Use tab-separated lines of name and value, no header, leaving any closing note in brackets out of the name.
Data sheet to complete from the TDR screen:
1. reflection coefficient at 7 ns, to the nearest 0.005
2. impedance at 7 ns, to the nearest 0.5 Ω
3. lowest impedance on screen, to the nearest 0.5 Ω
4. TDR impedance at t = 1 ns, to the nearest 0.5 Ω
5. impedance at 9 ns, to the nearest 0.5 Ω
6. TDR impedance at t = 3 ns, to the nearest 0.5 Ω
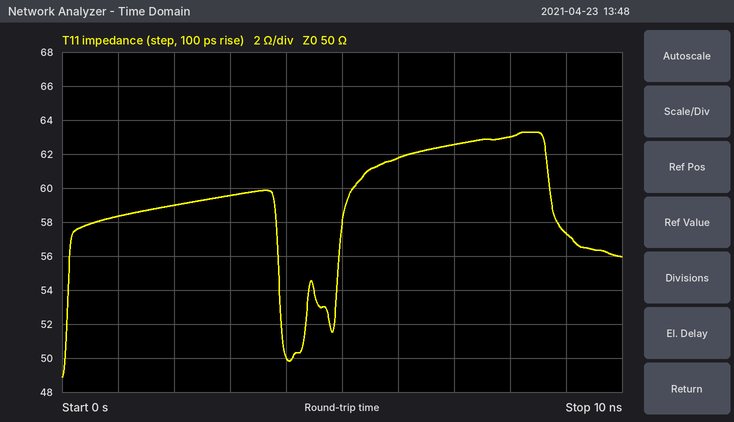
reflection coefficient at 7 ns, to the nearest 0.005	+0.110
impedance at 7 ns, to the nearest 0.5 Ω	62.5 Ω
lowest impedance on screen, to the nearest 0.5 Ω	49.0 Ω
TDR impedance at t = 1 ns, to the nearest 0.5 Ω	58.5 Ω
impedance at 9 ns, to the nearest 0.5 Ω	57.5 Ω
TDR impedance at t = 3 ns, to the nearest 0.5 Ω	59.5 Ω
